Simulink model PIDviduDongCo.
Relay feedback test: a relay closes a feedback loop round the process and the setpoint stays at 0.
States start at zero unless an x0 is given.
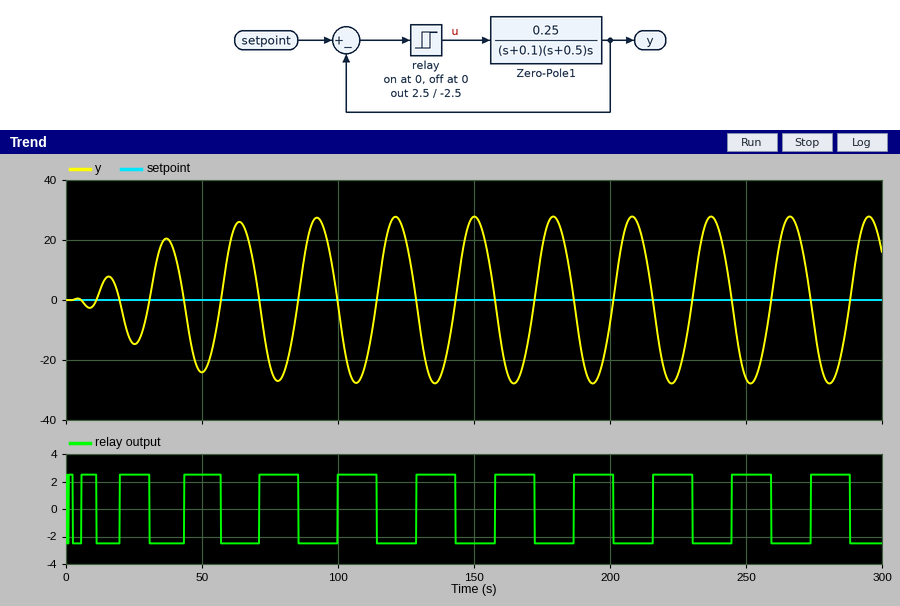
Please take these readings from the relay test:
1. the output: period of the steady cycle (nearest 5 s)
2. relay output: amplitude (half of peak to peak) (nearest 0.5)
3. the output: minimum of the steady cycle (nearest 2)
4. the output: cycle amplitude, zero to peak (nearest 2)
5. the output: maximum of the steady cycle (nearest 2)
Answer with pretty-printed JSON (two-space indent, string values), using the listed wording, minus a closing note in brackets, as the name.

{
  "the output: period of the steady cycle": "30 s",
  "relay output: amplitude (half of peak to peak)": "2.5",
  "the output: minimum of the steady cycle": "-28",
  "the output: cycle amplitude, zero to peak": "28",
  "the output: maximum of the steady cycle": "28"
}
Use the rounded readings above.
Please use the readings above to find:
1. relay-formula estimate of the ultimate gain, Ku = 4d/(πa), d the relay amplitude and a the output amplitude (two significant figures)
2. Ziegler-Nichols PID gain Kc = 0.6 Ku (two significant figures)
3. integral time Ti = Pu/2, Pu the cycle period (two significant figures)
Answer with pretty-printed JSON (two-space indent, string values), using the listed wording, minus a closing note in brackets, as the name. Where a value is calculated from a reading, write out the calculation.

{
  "relay-formula estimate of the ultimate gain, Ku = 4d/(πa), d the relay amplitude and a the output amplitude": "4 × 2.5 / (π × 28) = 0.11",
  "Ziegler-Nichols PID gain Kc = 0.6 Ku": "0.6 × 0.11 = 0.066",
  "integral time Ti = Pu/2, Pu the cycle period": "30 / 2 = 15 s"
}
